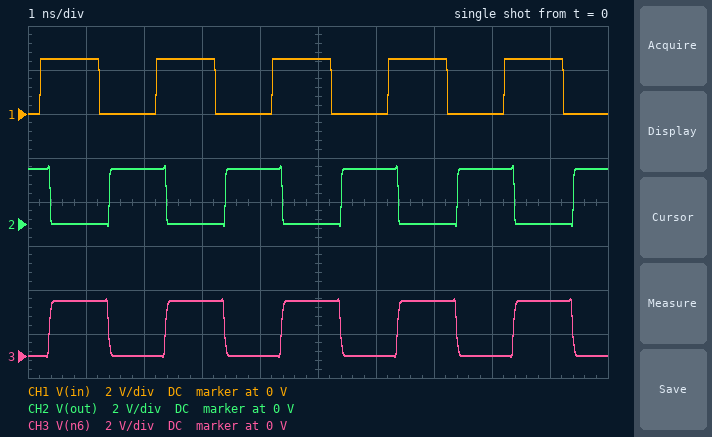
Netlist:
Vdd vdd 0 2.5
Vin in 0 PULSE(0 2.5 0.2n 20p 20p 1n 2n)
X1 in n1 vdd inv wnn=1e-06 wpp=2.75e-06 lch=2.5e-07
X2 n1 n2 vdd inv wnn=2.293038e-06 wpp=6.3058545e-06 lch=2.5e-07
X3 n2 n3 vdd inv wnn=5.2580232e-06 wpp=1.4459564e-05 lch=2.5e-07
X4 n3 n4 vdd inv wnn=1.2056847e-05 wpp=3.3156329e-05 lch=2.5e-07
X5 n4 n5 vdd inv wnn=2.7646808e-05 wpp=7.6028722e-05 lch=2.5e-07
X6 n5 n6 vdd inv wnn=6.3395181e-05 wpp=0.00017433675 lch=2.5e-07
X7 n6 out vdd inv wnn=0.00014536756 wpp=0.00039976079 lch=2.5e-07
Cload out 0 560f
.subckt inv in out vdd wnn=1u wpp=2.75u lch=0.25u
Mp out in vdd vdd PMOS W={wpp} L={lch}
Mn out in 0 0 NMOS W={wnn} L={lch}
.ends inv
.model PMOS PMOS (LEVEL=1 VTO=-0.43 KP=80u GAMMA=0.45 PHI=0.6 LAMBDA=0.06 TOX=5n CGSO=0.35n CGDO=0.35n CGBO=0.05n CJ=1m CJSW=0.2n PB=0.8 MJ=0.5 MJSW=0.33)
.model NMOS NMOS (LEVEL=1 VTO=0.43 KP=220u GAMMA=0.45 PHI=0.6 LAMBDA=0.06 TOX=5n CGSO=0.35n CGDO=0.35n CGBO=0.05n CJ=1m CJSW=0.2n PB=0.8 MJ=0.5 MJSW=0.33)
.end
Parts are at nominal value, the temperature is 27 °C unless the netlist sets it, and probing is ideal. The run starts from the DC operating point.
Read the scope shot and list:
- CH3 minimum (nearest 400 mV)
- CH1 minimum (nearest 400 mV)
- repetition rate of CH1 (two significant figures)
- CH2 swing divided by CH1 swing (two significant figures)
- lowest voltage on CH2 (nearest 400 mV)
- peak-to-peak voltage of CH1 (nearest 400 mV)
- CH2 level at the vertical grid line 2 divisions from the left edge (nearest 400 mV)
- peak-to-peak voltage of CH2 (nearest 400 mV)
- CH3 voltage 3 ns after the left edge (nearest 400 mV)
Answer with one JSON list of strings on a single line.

["0 V", "0 V", "500 MHz", "1.1", "0 V", "2.4 V", "2.4 V", "2.8 V", "2.4 V"]
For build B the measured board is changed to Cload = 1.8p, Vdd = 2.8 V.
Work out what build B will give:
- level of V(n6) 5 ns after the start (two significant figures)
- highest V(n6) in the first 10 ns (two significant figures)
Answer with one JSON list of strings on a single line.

["2.8 V", "2.9 V"]
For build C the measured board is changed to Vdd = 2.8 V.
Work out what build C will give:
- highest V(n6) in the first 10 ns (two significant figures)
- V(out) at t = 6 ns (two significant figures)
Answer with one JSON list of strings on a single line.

["2.9 V", "2.8 V"]
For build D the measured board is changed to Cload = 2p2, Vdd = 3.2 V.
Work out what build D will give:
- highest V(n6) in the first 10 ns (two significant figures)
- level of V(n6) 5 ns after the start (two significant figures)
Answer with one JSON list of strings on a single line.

["3.3 V", "3.2 V"]
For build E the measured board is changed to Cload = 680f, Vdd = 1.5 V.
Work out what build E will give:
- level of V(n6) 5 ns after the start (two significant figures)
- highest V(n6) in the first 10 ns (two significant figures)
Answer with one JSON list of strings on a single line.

["1.5 V", "1.6 V"]
